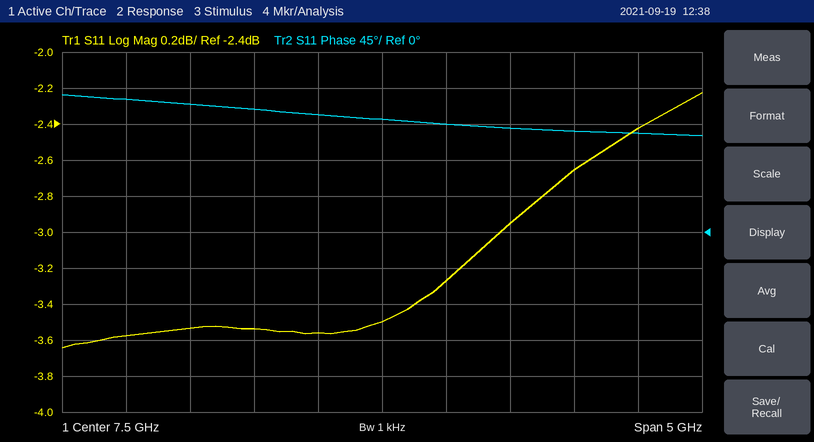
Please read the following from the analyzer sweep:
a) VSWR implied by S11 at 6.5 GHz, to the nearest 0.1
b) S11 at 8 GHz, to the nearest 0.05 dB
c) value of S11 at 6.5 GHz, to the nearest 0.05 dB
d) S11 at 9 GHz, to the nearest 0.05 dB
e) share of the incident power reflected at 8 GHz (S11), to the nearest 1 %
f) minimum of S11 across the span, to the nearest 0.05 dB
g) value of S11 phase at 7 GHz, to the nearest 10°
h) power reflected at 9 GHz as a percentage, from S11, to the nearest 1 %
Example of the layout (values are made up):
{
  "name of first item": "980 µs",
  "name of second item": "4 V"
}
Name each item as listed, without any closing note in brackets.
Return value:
{
  "VSWR implied by S11 at 6.5 GHz, to the nearest 0.1": "5.0",
  "S11 at 8 GHz, to the nearest 0.05 dB": "-3.25 dB",
  "value of S11 at 6.5 GHz, to the nearest 0.05 dB": "-3.55 dB",
  "S11 at 9 GHz, to the nearest 0.05 dB": "-2.65 dB",
  "share of the incident power reflected at 8 GHz (S11), to the nearest 1 %": "47 %",
  "minimum of S11 across the span, to the nearest 0.05 dB": "-3.65 dB",
  "value of S11 phase at 7 GHz, to the nearest 10°": "150°",
  "power reflected at 9 GHz as a percentage, from S11, to the nearest 1 %": "54 %"
}
